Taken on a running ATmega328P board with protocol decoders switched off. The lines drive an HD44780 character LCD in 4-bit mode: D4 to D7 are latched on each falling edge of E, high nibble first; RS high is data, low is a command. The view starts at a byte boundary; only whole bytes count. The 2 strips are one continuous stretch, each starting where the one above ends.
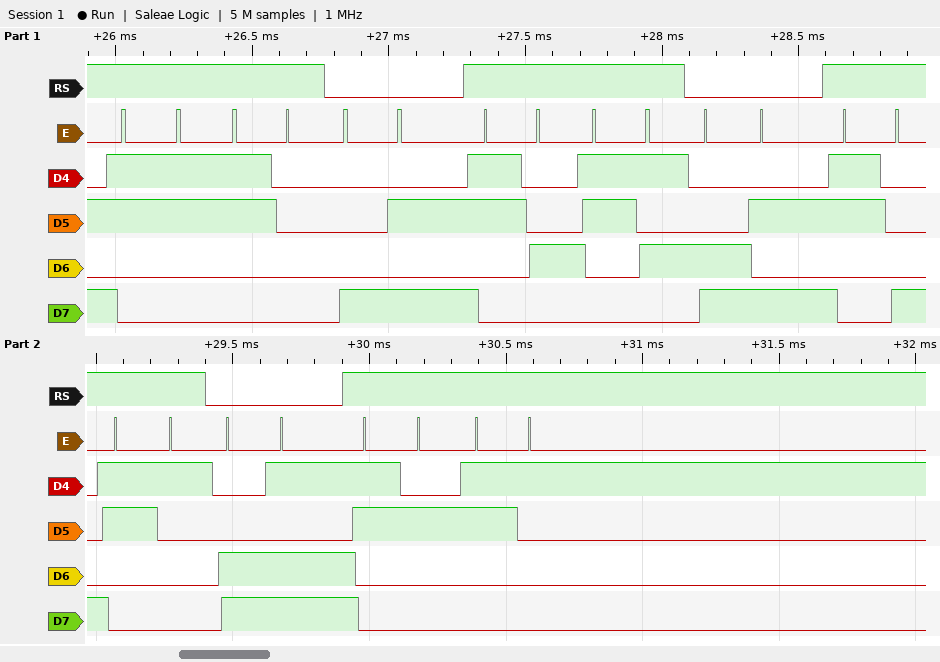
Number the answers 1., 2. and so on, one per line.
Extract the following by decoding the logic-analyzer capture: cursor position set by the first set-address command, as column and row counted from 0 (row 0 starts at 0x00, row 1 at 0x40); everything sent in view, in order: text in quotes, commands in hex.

1. column 10, row 0
2. "30" 0x8A "45" 0xCA "81" 0xCD "21"
